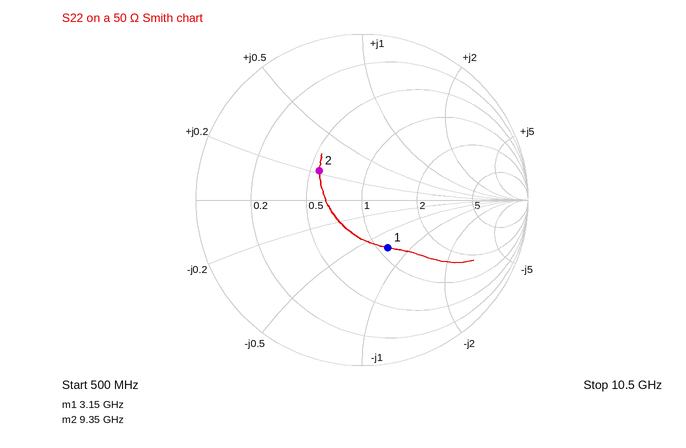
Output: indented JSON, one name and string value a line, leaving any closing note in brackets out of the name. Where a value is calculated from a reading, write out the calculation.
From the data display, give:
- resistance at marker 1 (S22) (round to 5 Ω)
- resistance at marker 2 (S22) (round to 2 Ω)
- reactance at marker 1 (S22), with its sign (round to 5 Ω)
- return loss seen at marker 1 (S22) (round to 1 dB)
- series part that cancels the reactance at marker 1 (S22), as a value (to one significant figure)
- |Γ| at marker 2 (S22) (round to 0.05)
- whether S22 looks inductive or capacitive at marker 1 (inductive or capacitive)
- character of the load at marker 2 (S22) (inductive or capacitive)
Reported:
{
  "resistance at marker 1 (S22)": "55 Ω",
  "resistance at marker 2 (S22)": "28 Ω",
  "reactance at marker 1 (S22), with its sign": "-35 Ω",
  "return loss seen at marker 1 (S22)": "10 dB",
  "series part that cancels the reactance at marker 1 (S22), as a value": "L = 35 Ω/(2π × 3.15 GHz) ≈ 2 nH",
  "|Γ| at marker 2 (S22)": "0.30",
  "whether S22 looks inductive or capacitive at marker 1": "capacitive",
  "character of the load at marker 2 (S22)": "inductive"
}
